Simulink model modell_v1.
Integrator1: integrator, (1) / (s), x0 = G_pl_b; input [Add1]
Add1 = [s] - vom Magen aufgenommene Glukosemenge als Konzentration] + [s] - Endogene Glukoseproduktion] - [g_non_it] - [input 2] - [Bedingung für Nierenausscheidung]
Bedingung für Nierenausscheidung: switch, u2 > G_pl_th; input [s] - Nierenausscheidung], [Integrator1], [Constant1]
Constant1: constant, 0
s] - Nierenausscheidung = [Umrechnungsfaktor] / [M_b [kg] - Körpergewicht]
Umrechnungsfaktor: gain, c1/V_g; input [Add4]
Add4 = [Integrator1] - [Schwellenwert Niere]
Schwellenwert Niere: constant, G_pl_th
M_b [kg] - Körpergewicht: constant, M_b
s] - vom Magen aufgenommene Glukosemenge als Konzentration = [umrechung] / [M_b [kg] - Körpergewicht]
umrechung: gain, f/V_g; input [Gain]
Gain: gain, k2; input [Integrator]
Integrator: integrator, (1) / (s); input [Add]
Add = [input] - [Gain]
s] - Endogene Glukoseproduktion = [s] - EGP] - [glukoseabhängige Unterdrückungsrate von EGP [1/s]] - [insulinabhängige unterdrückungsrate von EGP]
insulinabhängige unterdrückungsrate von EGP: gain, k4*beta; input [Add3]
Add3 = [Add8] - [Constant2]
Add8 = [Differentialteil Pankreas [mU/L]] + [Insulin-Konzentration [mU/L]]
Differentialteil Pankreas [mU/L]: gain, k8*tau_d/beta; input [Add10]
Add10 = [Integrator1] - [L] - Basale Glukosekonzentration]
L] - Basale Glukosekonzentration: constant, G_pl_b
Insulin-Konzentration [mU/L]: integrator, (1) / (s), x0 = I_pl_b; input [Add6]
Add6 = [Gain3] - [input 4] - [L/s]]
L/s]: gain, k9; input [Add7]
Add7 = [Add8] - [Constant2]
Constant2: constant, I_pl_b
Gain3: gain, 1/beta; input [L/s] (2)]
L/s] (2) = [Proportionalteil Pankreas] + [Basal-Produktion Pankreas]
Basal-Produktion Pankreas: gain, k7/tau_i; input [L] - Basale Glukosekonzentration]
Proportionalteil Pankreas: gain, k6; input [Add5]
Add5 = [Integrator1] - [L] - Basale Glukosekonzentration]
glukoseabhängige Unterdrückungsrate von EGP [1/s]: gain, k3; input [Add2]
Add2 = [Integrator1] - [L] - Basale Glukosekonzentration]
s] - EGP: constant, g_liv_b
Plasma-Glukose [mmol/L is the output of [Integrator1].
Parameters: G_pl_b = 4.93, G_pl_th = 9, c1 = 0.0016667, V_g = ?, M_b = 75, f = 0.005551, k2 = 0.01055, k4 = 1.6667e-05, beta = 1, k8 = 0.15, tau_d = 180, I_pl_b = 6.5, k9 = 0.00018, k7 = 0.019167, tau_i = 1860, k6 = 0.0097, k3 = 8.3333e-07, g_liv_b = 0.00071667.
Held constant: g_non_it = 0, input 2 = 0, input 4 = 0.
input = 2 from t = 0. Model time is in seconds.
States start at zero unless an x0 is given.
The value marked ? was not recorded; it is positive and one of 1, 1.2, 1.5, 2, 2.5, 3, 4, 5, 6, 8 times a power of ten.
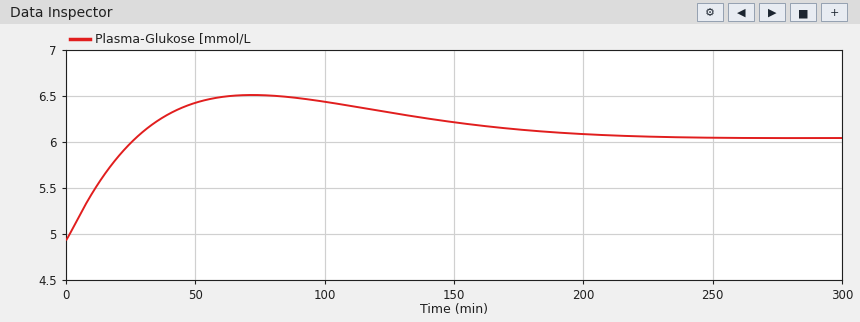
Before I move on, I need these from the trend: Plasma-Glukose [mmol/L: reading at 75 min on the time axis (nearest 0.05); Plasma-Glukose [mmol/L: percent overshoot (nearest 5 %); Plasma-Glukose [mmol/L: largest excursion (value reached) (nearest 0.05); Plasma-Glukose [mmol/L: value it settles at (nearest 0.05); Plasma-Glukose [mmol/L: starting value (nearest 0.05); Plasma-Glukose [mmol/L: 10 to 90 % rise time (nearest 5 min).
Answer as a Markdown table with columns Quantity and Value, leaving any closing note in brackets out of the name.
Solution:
| Quantity | Value |
|---|---|
| Plasma-Glukose [mmol/L: reading at 75 min on the time axis | 6.50 |
| Plasma-Glukose [mmol/L: percent overshoot | 40 % |
| Plasma-Glukose [mmol/L: largest excursion (value reached) | 6.50 |
| Plasma-Glukose [mmol/L: value it settles at | 6.05 |
| Plasma-Glukose [mmol/L: starting value | 4.95 |
| Plasma-Glukose [mmol/L: 10 to 90 % rise time | 20 min |
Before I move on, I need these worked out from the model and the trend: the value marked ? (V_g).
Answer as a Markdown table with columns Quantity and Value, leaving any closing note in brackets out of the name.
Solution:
| Quantity | Value |
|---|---|
| the value marked ? | 0.5 |
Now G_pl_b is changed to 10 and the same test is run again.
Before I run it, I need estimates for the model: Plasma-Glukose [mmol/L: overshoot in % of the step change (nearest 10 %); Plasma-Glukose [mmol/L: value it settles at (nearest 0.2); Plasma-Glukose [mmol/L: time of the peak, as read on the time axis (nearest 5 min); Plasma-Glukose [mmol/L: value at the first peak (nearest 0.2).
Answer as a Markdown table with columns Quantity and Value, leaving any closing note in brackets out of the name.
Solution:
| Quantity | Value |
|---|---|
| Plasma-Glukose [mmol/L: overshoot in % of the step change | 40 % |
| Plasma-Glukose [mmol/L: value it settles at | 11.0 |
| Plasma-Glukose [mmol/L: time of the peak, as read on the time axis | 70 min |
| Plasma-Glukose [mmol/L: value at the first peak | 11.4 |
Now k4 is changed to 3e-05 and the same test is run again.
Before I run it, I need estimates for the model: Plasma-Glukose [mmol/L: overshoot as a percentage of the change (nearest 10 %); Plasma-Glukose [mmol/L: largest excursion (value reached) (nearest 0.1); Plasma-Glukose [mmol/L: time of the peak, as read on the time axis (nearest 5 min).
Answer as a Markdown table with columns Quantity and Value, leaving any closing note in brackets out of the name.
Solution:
| Quantity | Value |
|---|---|
| Plasma-Glukose [mmol/L: overshoot as a percentage of the change | 50 % |
| Plasma-Glukose [mmol/L: largest excursion (value reached) | 5.9 |
| Plasma-Glukose [mmol/L: time of the peak, as read on the time axis | 45 min |
